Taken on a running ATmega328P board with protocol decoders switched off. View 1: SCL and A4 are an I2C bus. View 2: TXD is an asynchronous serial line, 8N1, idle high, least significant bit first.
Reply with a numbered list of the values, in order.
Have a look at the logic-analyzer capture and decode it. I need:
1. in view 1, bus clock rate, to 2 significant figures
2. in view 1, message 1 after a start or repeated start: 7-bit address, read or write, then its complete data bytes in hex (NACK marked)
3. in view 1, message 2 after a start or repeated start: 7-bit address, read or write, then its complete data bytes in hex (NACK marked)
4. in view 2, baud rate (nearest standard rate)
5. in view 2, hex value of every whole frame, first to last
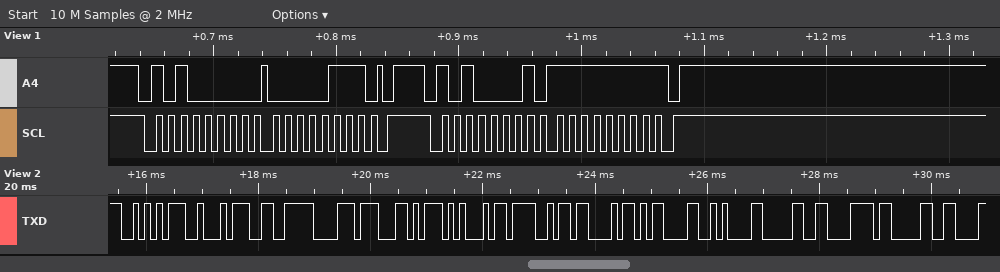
1. 100 kHz
2. 0x50 write: 07
3. 0x50 read: FF NACK
4. 9600 baud
5. 0xAA 0xA2 0xE6 0xB8 0xAC 0x45 0x4F 0x43 0x0D 0x0A 0x30 0x78 0x30
